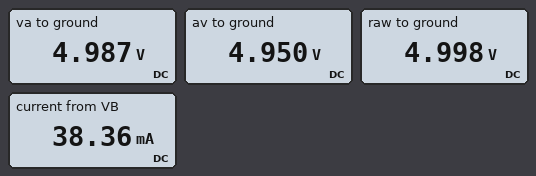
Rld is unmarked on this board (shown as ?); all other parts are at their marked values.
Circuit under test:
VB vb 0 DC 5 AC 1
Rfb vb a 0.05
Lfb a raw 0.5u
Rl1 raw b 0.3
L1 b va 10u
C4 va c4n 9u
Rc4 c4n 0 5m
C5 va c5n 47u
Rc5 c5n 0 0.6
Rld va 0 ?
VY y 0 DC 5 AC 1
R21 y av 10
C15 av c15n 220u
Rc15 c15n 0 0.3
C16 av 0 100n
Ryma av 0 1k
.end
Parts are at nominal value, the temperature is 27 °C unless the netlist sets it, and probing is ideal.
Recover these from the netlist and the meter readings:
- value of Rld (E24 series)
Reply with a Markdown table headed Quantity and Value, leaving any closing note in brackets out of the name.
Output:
| Quantity | Value |
|---|---|
| value of Rld | 130 Ω |
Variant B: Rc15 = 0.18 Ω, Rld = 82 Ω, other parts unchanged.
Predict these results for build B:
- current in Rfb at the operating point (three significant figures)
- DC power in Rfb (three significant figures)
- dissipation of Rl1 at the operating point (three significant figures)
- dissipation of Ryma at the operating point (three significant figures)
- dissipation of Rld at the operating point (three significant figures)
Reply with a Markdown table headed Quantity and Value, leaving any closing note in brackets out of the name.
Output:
| Quantity | Value |
|---|---|
| current in Rfb at the operating point | 60.7 mA |
| DC power in Rfb | 184 µW |
| dissipation of Rl1 at the operating point | 1.11 mW |
| dissipation of Ryma at the operating point | 24.5 mW |
| dissipation of Rld at the operating point | 302 mW |
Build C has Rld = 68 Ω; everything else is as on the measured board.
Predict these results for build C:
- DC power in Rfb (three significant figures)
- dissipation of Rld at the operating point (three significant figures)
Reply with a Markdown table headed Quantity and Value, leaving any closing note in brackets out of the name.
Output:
| Quantity | Value |
|---|---|
| DC power in Rfb | 268 µW |
| dissipation of Rld at the operating point | 364 mW |
